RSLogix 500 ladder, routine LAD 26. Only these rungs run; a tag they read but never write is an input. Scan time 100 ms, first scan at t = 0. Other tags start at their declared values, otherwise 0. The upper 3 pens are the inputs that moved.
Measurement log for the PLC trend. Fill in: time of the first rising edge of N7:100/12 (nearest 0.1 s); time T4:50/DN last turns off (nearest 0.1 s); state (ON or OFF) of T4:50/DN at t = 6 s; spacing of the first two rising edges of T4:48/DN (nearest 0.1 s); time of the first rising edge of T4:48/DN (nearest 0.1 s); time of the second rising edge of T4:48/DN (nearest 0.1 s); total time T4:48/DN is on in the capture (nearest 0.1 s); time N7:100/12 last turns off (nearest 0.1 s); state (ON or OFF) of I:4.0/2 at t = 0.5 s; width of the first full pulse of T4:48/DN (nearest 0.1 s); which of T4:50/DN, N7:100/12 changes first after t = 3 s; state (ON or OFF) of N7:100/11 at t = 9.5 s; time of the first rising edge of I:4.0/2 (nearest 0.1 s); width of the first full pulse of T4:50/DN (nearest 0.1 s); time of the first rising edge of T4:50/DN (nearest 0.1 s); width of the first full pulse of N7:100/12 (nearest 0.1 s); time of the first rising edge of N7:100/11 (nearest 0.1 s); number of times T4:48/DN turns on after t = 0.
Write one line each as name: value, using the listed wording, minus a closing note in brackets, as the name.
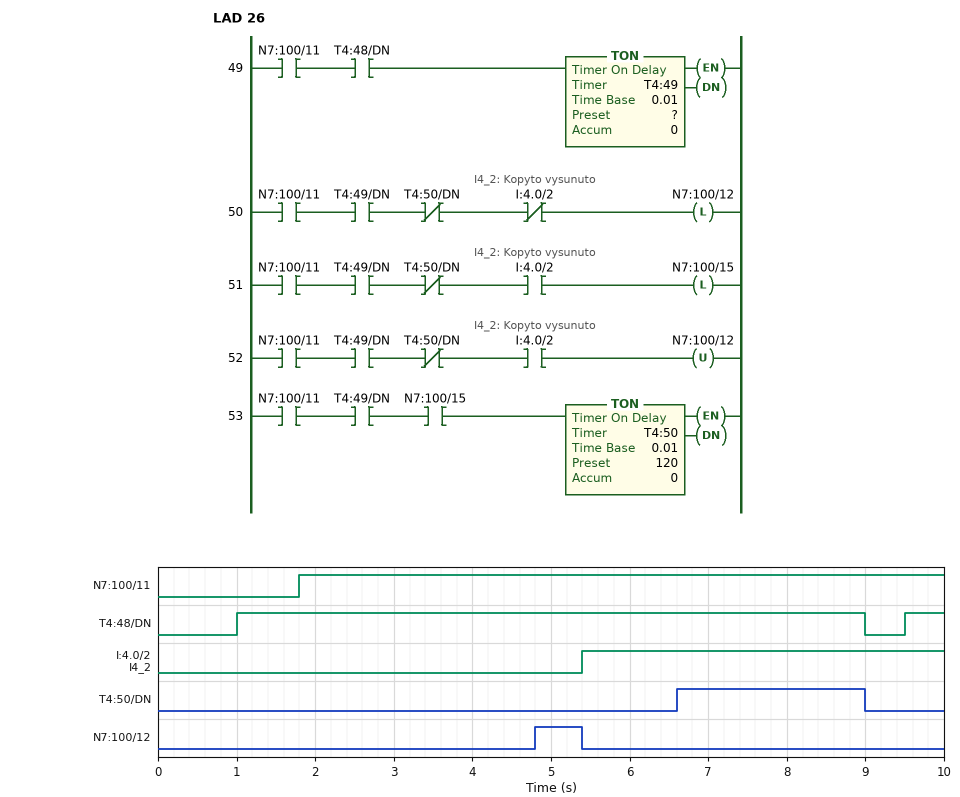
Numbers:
time of the first rising edge of N7:100/12: 4.8 s
time T4:50/DN last turns off: 9.0 s
state (ON or OFF) of T4:50/DN at t = 6 s: OFF
spacing of the first two rising edges of T4:48/DN: 8.5 s
time of the first rising edge of T4:48/DN: 1.0 s
time of the second rising edge of T4:48/DN: 9.5 s
total time T4:48/DN is on in the capture: 8.5 s
time N7:100/12 last turns off: 5.4 s
state (ON or OFF) of I:4.0/2 at t = 0.5 s: OFF
width of the first full pulse of T4:48/DN: 8.0 s
which of T4:50/DN, N7:100/12 changes first after t = 3 s: N7:100/12
state (ON or OFF) of N7:100/11 at t = 9.5 s: ON
time of the first rising edge of I:4.0/2: 5.4 s
width of the first full pulse of T4:50/DN: 2.4 s
time of the first rising edge of T4:50/DN: 6.6 s
width of the first full pulse of N7:100/12: 0.6 s
time of the first rising edge of N7:100/11: 1.8 s
number of times T4:48/DN turns on after t = 0: 2
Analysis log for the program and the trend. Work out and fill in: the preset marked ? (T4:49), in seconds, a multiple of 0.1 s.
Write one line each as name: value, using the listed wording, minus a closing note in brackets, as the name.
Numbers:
the preset marked ? (T4:49), in seconds, a multiple of 0.1 s: 3.0 s
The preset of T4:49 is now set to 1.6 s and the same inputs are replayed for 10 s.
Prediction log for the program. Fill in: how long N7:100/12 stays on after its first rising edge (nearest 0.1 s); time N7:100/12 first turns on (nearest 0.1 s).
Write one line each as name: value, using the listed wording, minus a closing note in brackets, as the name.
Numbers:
how long N7:100/12 stays on after its first rising edge: 2.0 s
time N7:100/12 first turns on: 3.4 s
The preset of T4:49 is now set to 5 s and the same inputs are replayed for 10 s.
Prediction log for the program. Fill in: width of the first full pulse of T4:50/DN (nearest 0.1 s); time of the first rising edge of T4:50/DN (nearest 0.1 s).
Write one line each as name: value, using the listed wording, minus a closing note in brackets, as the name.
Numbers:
width of the first full pulse of T4:50/DN: 1.0 s
time of the first rising edge of T4:50/DN: 8.0 s
